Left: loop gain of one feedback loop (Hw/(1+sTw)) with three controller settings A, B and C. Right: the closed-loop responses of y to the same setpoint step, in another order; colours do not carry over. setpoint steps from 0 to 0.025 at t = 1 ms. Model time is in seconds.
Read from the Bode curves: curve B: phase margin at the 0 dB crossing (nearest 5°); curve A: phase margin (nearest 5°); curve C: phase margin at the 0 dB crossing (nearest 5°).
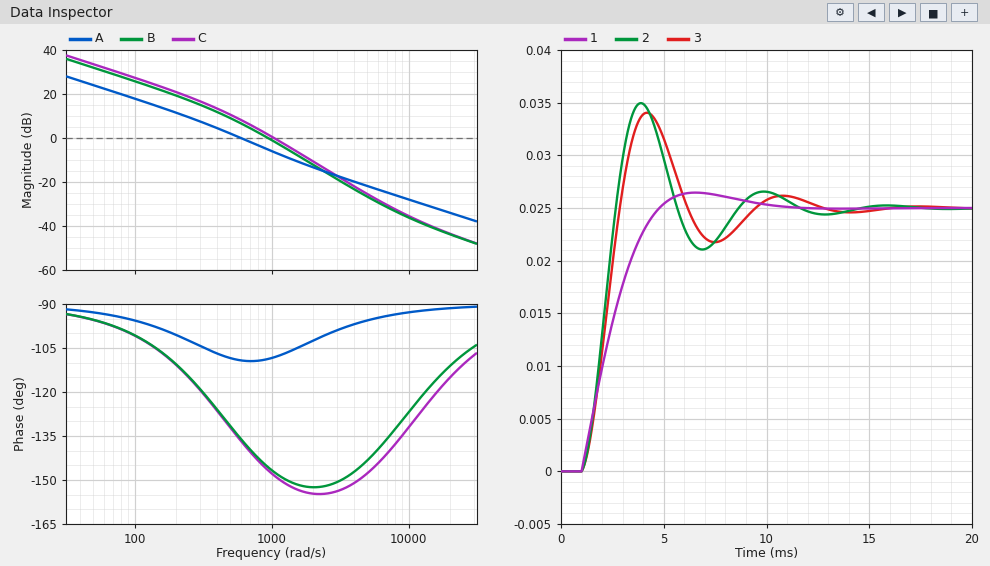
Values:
35°
70°
30°
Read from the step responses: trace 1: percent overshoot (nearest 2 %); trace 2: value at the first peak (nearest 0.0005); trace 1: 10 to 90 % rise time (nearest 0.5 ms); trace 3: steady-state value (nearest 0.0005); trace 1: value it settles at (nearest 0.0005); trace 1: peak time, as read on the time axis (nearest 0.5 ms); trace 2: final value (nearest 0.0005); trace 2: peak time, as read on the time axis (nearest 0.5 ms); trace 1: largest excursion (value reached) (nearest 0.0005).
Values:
6 %
0.0350
2.5 ms
0.0250
0.0250
6.5 ms
0.0250
4.0 ms
0.0265
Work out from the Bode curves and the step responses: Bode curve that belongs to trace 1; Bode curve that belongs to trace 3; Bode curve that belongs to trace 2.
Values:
A
B
C
